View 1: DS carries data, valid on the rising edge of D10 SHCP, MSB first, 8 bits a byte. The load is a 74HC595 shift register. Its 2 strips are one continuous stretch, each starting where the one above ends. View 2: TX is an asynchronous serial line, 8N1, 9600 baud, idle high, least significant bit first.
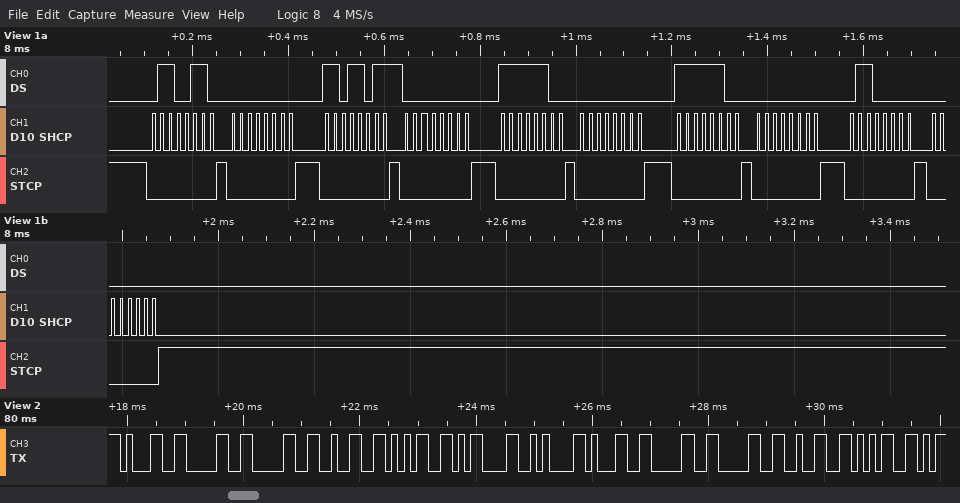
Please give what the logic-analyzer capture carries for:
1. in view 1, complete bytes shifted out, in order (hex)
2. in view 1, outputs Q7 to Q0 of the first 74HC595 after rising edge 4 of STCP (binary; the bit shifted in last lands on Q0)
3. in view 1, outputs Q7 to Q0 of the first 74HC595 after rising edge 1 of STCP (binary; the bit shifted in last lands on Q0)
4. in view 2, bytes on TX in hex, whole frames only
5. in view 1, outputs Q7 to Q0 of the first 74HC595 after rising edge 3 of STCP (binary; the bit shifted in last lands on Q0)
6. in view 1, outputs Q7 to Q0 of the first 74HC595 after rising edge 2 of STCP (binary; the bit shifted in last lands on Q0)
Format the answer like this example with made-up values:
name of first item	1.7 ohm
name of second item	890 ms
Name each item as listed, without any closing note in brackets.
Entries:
in view 1, complete bytes shifted out, in order	66 00 DB 00 FC 00 FC 00 60 00
in view 1, outputs Q7 to Q0 of the first 74HC595 after rising edge 4 of STCP	00000000
in view 1, outputs Q7 to Q0 of the first 74HC595 after rising edge 1 of STCP	01100110
in view 2, bytes on TX in hex, whole frames only	0x31 0x30 0x30 0x32 0x35 0x0D 0x0A 0x31 0x30 0x30 0x32 0x35
in view 1, outputs Q7 to Q0 of the first 74HC595 after rising edge 3 of STCP	11011011
in view 1, outputs Q7 to Q0 of the first 74HC595 after rising edge 2 of STCP	00000000
